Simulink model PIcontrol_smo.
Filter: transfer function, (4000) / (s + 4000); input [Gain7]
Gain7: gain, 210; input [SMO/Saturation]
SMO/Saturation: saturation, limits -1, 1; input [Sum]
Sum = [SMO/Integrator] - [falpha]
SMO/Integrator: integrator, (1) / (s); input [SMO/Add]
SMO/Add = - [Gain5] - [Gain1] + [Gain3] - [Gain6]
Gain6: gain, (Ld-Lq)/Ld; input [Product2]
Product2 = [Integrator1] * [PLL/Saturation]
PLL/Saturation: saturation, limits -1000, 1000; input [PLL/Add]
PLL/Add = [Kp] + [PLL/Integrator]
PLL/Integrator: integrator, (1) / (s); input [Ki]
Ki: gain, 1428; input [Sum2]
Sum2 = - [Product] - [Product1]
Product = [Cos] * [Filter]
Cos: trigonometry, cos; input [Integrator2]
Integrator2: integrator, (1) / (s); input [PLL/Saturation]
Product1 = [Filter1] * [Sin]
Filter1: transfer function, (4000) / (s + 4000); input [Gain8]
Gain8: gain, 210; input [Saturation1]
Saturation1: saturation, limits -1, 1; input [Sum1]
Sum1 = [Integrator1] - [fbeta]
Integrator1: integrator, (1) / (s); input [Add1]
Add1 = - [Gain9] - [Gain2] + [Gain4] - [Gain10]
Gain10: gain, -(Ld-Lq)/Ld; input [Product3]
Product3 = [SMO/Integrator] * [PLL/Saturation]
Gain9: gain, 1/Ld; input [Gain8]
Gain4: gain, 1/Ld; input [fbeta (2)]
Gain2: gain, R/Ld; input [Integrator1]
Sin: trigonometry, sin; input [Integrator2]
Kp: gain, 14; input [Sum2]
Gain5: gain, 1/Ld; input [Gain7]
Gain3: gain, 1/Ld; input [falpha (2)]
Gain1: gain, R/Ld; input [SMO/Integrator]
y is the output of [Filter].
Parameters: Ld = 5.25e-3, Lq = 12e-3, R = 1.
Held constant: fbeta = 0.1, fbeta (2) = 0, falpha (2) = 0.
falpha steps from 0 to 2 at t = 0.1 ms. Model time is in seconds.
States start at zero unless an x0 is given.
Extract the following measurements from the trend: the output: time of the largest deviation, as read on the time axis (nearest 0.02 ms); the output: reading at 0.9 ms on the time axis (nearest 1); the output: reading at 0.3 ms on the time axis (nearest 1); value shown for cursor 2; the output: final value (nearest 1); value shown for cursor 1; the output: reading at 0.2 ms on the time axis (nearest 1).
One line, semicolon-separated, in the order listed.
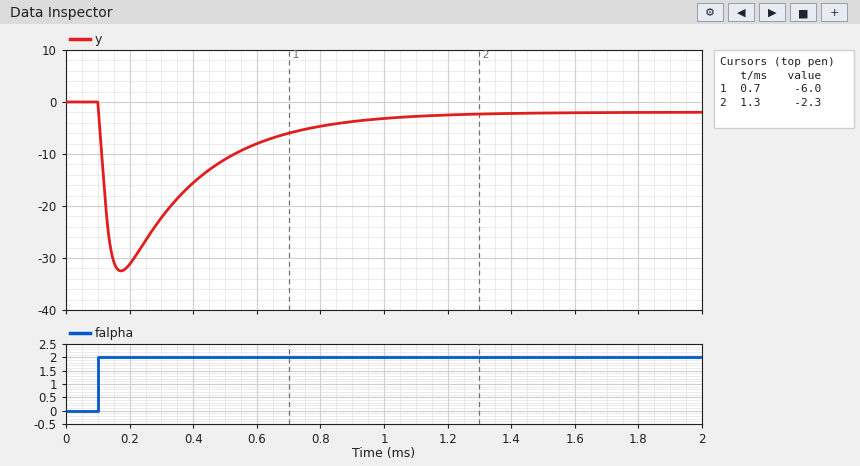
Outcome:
0.18 ms; -4; -22; -2.3; -2; -6.0; -31
